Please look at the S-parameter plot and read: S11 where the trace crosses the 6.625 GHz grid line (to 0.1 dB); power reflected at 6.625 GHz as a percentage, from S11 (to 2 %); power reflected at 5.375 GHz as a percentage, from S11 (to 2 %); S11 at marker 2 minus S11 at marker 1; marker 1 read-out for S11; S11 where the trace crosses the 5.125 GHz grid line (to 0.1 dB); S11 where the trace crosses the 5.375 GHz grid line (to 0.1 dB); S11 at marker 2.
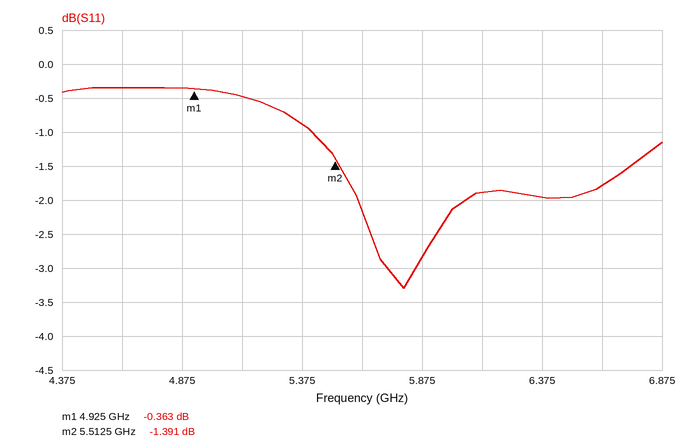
-1.8 dB
66 %
82 %
-1.028 dB
-0.363 dB
-0.5 dB
-0.9 dB
-1.391 dB
